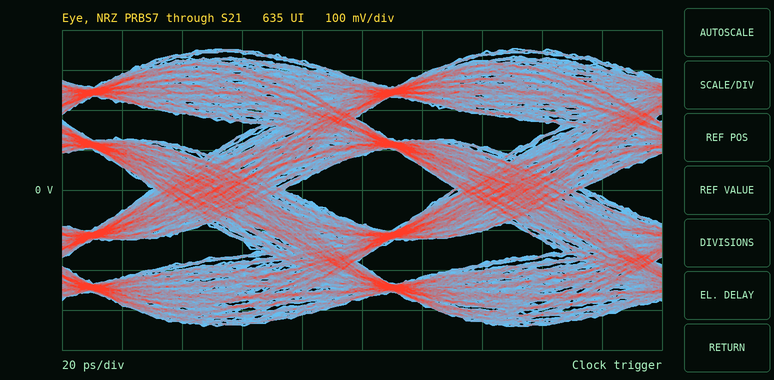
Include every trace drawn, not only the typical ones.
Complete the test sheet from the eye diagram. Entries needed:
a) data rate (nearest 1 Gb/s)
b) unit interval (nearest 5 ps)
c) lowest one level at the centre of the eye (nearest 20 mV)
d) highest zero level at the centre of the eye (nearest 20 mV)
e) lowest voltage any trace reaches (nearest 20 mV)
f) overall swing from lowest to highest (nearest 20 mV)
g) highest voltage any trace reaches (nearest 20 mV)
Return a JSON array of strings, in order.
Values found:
["10 Gb/s", "100 ps", "80 mV", "-80 mV", "-340 mV", "700 mV", "360 mV"]
